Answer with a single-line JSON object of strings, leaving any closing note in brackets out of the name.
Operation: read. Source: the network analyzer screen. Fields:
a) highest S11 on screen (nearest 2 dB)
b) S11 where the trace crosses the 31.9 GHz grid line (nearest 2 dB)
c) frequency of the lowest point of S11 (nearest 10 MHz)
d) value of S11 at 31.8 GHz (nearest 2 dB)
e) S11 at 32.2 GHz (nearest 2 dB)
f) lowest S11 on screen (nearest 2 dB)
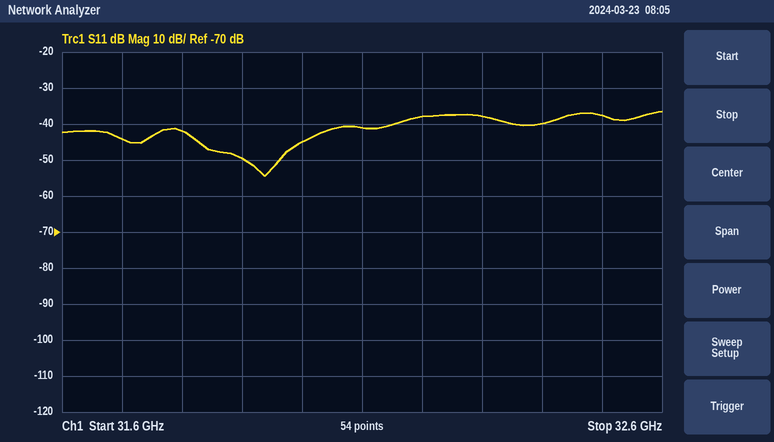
{"highest S11 on screen": "-36 dB", "S11 where the trace crosses the 31.9 GHz grid line": "-50 dB", "frequency of the lowest point of S11": "31.94 GHz", "value of S11 at 31.8 GHz": "-42 dB", "S11 at 32.2 GHz": "-38 dB", "lowest S11 on screen": "-54 dB"}
